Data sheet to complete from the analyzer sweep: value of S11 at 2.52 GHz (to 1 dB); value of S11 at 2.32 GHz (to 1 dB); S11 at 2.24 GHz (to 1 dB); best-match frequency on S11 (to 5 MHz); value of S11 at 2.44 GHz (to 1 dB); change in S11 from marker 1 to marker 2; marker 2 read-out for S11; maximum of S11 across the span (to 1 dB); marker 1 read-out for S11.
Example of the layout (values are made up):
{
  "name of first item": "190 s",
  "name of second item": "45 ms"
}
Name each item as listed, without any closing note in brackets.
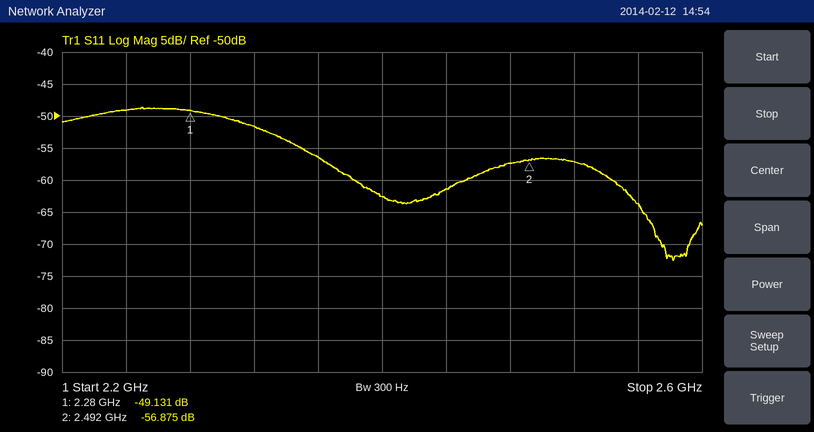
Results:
{
  "value of S11 at 2.52 GHz": "-57 dB",
  "value of S11 at 2.32 GHz": "-52 dB",
  "S11 at 2.24 GHz": "-49 dB",
  "best-match frequency on S11": "2.580 GHz",
  "value of S11 at 2.44 GHz": "-61 dB",
  "change in S11 from marker 1 to marker 2": "-7.744 dB",
  "marker 2 read-out for S11": "-56.875 dB",
  "maximum of S11 across the span": "-49 dB",
  "marker 1 read-out for S11": "-49.131 dB"
}
